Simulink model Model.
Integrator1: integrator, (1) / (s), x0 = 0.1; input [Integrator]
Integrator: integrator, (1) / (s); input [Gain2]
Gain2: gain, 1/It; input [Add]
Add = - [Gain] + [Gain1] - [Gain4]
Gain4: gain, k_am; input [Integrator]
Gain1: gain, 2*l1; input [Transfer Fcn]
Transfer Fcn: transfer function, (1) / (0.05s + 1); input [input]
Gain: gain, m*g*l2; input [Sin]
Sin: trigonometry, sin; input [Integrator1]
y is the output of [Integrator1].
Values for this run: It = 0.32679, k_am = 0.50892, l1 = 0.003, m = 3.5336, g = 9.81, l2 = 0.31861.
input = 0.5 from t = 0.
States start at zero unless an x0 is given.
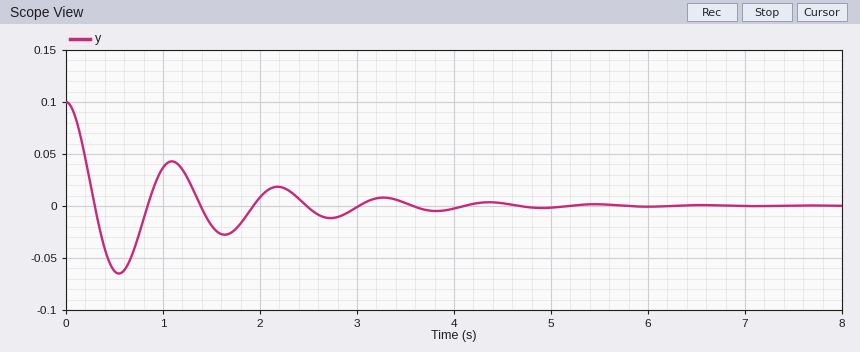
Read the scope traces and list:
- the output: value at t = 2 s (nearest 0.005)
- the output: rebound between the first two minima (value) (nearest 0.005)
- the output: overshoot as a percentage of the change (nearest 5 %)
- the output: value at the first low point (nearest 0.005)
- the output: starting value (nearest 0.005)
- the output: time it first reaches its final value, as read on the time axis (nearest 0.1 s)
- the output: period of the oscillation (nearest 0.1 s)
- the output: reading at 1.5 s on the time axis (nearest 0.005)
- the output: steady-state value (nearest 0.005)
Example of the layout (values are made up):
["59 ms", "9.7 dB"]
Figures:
["0.010", "0.045", "65 %", "-0.065", "0.100", "0.3 s", "1.1 s", "-0.020", "0.000"]
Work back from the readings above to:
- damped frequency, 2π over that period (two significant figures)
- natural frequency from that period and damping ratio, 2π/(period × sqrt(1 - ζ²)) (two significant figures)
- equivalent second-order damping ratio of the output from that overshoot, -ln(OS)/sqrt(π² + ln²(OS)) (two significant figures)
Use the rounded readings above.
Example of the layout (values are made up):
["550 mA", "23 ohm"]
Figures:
["5.7 rad/s", "5.8 rad/s", "0.14"]
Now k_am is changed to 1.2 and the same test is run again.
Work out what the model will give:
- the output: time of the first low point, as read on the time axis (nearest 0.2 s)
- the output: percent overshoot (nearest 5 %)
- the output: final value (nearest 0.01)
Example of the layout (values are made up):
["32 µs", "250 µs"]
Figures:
["0.6 s", "35 %", "0.00"]
